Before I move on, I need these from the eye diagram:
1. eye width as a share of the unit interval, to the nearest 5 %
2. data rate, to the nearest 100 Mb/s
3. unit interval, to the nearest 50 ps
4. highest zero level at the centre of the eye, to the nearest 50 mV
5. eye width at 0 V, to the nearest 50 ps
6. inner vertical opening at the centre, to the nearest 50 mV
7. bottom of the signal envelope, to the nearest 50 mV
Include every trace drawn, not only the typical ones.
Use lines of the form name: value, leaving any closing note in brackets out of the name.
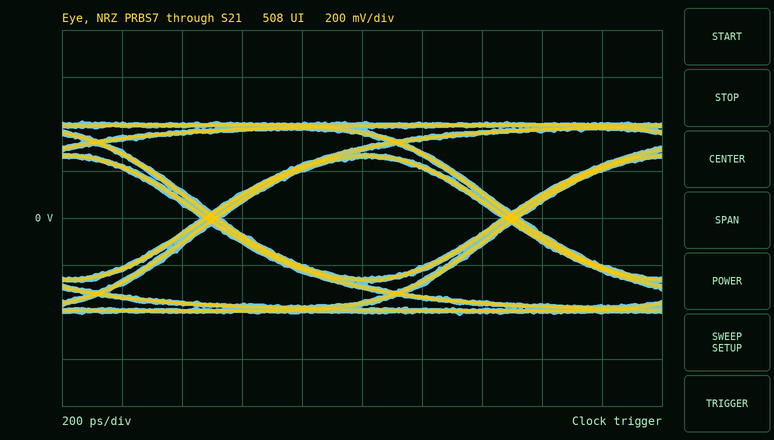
eye width as a share of the unit interval, to the nearest 5 %: 95 %
data rate, to the nearest 100 Mb/s: 1.0 Gb/s
unit interval, to the nearest 50 ps: 1.00 ns
highest zero level at the centre of the eye, to the nearest 50 mV: -250 mV
eye width at 0 V, to the nearest 50 ps: 950 ps
inner vertical opening at the centre, to the nearest 50 mV: 500 mV
bottom of the signal envelope, to the nearest 50 mV: -400 mV
